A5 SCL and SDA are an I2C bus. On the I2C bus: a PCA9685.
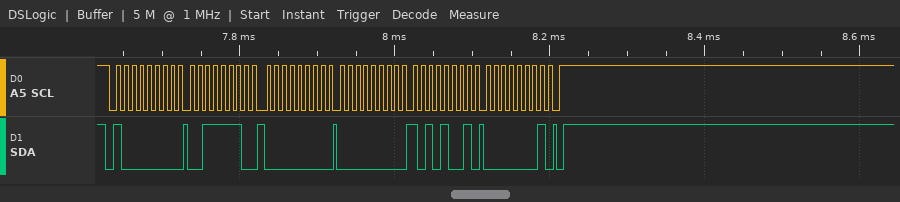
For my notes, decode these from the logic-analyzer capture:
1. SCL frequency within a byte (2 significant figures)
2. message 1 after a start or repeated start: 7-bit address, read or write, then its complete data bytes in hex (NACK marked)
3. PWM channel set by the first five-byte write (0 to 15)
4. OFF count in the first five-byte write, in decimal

100 kHz
0x40 write: 3E 00 00 A9 01
14
425
